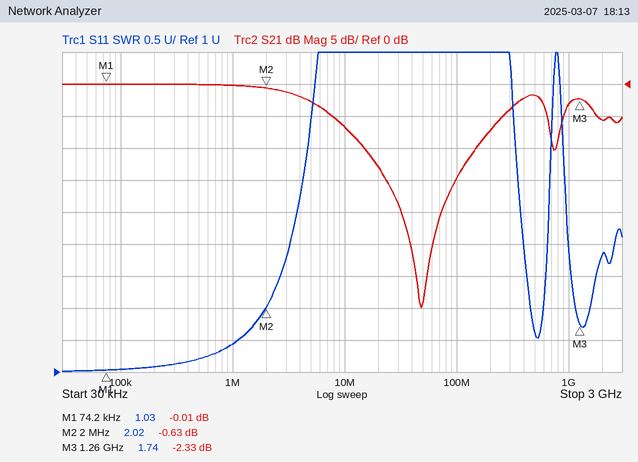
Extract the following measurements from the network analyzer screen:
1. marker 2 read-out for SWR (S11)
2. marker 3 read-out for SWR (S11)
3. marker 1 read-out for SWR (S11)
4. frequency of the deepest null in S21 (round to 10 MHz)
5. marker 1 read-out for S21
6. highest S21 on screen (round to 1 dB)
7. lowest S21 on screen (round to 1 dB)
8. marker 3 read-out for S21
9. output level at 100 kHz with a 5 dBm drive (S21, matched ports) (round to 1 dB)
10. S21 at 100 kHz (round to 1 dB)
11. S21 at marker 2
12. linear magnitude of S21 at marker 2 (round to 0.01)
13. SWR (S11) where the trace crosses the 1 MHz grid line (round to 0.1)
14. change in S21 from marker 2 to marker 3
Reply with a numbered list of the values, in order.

1. 2.02
2. 1.74
3. 1.03
4. 50 MHz
5. -0.01 dB
6. 0 dB
7. -35 dB
8. -2.33 dB
9. 5 dBm
10. 0 dB
11. -0.63 dB
12. 0.93
13. 1.4
14. -1.70 dB
